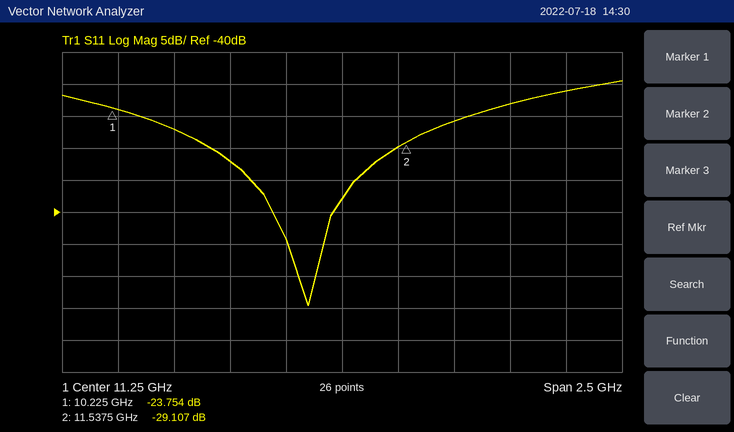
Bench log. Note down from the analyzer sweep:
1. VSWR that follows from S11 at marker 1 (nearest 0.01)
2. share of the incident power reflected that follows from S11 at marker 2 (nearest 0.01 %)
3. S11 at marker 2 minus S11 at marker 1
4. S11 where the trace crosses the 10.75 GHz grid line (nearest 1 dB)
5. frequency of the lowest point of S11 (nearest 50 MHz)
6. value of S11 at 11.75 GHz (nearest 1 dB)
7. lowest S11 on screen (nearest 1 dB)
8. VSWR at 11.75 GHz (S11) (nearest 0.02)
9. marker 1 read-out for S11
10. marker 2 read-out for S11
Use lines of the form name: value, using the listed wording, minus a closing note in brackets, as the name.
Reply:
VSWR that follows from S11 at marker 1: 1.14
share of the incident power reflected that follows from S11 at marker 2: 0.12 %
S11 at marker 2 minus S11 at marker 1: -5.353 dB
S11 where the trace crosses the 10.75 GHz grid line: -32 dB
frequency of the lowest point of S11: 11.10 GHz
value of S11 at 11.75 GHz: -26 dB
lowest S11 on screen: -55 dB
VSWR at 11.75 GHz (S11): 1.10
marker 1 read-out for S11: -23.754 dB
marker 2 read-out for S11: -29.107 dB
